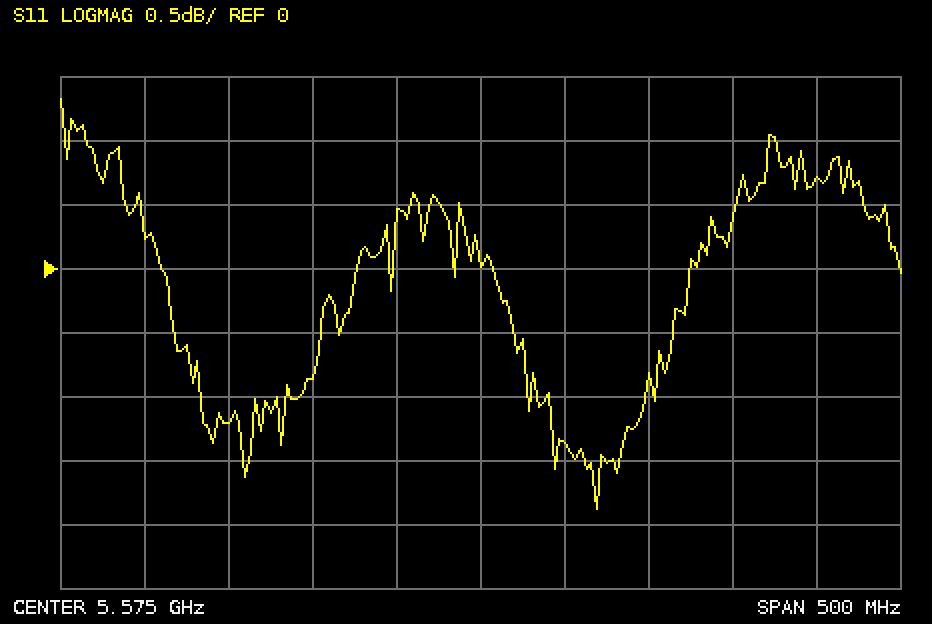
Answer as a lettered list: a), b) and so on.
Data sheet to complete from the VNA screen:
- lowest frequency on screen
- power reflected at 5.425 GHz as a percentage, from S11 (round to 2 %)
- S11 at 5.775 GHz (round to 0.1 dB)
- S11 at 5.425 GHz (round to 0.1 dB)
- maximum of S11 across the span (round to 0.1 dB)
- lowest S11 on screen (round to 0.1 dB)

a) 5.325 GHz
b) 76 %
c) 0.7 dB
d) -1.2 dB
e) 1.3 dB
f) -1.9 dB
